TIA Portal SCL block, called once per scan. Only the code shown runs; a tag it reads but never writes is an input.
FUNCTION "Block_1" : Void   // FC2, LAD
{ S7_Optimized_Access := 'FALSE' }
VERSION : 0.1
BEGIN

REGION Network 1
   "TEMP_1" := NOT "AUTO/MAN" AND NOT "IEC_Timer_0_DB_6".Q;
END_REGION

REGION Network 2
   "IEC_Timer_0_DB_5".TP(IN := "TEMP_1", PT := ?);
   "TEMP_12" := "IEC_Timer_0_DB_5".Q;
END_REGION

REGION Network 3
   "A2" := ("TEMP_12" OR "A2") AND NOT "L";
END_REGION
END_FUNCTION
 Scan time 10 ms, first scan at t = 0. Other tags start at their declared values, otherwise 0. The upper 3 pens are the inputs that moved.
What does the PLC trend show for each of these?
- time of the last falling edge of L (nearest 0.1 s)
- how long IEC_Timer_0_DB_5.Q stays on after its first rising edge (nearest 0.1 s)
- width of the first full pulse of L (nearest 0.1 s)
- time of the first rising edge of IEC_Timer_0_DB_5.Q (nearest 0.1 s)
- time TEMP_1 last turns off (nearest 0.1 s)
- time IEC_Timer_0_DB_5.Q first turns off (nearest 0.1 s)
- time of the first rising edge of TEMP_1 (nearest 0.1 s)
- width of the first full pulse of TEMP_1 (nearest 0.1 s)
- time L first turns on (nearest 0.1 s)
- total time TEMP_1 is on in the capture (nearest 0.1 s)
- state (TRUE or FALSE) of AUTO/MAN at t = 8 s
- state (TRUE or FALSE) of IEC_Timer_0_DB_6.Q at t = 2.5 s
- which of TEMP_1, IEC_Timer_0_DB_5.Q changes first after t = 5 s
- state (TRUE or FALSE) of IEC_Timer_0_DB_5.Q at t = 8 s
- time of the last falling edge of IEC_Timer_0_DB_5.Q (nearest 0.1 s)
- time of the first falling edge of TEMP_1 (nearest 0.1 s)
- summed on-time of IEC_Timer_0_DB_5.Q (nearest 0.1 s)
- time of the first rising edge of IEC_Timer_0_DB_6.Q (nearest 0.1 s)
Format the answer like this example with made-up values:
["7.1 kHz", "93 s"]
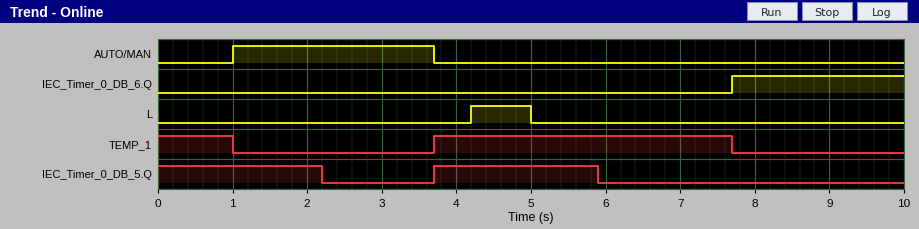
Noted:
["5.0 s", "2.2 s", "0.8 s", "3.7 s", "7.7 s", "2.2 s", "3.7 s", "4.0 s", "4.2 s", "5.0 s", "FALSE", "FALSE", "IEC_Timer_0_DB_5.Q", "FALSE", "5.9 s", "1.0 s", "4.4 s", "7.7 s"]
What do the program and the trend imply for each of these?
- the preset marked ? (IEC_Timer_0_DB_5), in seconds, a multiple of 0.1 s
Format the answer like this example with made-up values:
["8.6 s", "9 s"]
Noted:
["2.2 s"]
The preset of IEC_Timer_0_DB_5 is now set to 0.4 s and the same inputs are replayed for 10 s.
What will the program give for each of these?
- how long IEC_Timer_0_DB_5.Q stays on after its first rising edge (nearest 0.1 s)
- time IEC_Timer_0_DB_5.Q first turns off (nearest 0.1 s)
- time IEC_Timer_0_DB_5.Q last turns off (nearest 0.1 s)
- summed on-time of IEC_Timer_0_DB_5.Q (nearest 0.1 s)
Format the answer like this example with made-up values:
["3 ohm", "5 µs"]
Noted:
["0.4 s", "0.4 s", "4.1 s", "0.8 s"]
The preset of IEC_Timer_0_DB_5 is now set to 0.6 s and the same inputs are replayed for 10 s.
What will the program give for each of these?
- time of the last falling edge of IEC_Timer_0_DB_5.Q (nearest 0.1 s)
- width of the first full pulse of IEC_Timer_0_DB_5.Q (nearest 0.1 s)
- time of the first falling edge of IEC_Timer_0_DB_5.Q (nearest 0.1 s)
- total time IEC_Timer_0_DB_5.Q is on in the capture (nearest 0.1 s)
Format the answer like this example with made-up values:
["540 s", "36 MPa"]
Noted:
["4.3 s", "0.6 s", "0.6 s", "1.2 s"]
